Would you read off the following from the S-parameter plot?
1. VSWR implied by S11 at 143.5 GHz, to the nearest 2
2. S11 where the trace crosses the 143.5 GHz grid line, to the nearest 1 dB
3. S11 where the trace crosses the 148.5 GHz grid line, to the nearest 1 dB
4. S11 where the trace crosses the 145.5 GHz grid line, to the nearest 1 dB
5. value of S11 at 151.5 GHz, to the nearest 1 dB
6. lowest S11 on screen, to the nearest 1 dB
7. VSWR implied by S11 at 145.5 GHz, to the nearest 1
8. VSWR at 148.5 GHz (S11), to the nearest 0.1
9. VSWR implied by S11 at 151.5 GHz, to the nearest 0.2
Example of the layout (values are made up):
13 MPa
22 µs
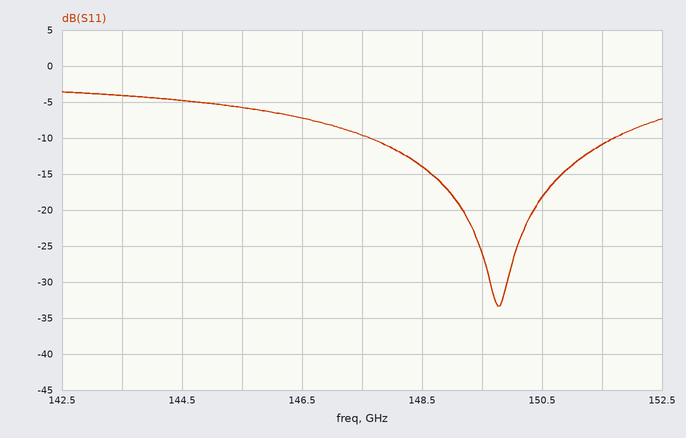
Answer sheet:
4
-4 dB
-14 dB
-6 dB
-11 dB
-33 dB
3
1.5
1.8
